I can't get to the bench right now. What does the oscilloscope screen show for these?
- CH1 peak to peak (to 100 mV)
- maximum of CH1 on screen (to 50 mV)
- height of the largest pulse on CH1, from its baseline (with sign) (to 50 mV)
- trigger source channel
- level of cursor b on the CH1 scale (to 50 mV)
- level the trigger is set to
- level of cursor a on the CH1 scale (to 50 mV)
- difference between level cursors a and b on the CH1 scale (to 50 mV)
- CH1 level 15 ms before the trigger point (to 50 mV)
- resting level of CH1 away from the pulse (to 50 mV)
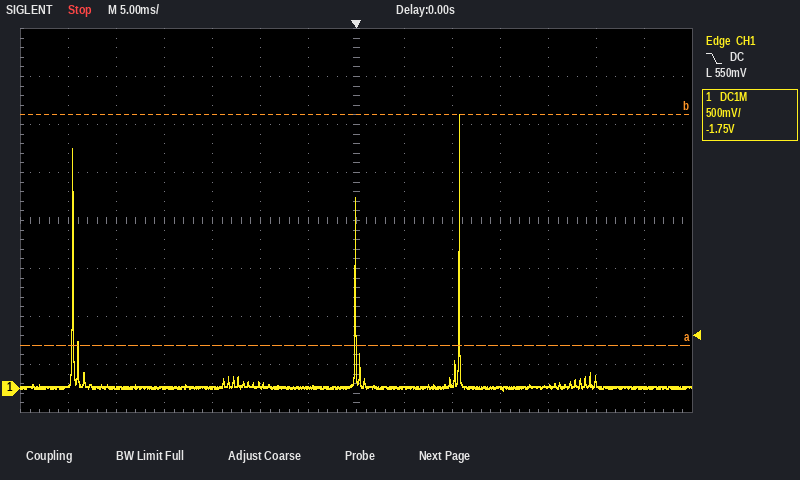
2.90 V
2.85 V
+2.85 V
CH1
2.85 V
550 mV
450 mV
2.40 V
0 mV
0 mV
